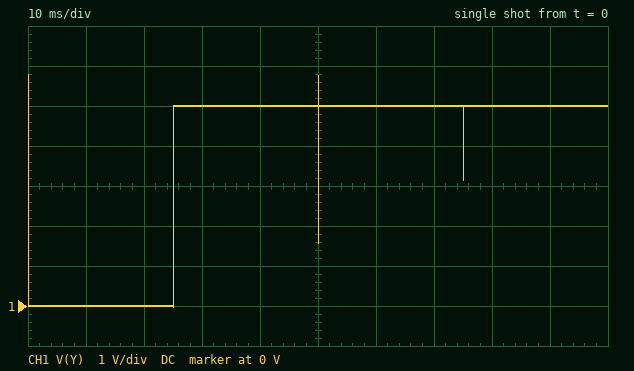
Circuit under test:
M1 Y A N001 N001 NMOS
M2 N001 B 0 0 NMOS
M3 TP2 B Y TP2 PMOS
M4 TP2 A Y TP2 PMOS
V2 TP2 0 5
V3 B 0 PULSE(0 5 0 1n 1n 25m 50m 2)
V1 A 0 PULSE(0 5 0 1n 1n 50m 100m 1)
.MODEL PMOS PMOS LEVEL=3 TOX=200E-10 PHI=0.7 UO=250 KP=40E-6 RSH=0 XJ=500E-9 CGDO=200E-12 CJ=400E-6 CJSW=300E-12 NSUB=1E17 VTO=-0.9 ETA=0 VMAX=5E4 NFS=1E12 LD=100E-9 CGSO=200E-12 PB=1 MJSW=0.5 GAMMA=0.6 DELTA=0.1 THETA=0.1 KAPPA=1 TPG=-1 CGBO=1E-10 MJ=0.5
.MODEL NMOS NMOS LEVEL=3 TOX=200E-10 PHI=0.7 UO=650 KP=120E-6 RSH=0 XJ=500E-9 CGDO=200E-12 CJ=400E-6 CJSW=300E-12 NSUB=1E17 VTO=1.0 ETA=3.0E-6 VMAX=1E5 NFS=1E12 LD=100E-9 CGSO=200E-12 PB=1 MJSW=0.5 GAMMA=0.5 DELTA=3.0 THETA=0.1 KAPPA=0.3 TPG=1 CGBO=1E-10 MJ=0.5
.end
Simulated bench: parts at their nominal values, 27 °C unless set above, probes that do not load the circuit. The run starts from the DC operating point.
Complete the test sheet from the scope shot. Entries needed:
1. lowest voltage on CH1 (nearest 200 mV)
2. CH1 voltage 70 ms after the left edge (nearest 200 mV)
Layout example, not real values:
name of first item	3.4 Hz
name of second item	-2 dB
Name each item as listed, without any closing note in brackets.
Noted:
lowest voltage on CH1	0 V
CH1 voltage 70 ms after the left edge	5.0 V
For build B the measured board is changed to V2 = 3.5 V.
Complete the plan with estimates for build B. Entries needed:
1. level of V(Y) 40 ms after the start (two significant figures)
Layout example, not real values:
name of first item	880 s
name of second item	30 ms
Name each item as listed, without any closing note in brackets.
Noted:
level of V(Y) 40 ms after the start	3.5 V
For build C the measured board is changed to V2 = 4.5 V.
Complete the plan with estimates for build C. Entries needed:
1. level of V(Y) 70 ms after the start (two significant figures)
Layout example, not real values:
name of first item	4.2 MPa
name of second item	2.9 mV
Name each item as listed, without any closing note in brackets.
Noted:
level of V(Y) 70 ms after the start	4.5 V
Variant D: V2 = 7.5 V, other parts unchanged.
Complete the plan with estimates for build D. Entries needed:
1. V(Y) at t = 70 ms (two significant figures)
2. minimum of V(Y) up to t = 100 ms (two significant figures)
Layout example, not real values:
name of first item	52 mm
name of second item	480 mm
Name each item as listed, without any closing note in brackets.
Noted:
V(Y) at t = 70 ms	7.5 V
minimum of V(Y) up to t = 100 ms	440 mV
